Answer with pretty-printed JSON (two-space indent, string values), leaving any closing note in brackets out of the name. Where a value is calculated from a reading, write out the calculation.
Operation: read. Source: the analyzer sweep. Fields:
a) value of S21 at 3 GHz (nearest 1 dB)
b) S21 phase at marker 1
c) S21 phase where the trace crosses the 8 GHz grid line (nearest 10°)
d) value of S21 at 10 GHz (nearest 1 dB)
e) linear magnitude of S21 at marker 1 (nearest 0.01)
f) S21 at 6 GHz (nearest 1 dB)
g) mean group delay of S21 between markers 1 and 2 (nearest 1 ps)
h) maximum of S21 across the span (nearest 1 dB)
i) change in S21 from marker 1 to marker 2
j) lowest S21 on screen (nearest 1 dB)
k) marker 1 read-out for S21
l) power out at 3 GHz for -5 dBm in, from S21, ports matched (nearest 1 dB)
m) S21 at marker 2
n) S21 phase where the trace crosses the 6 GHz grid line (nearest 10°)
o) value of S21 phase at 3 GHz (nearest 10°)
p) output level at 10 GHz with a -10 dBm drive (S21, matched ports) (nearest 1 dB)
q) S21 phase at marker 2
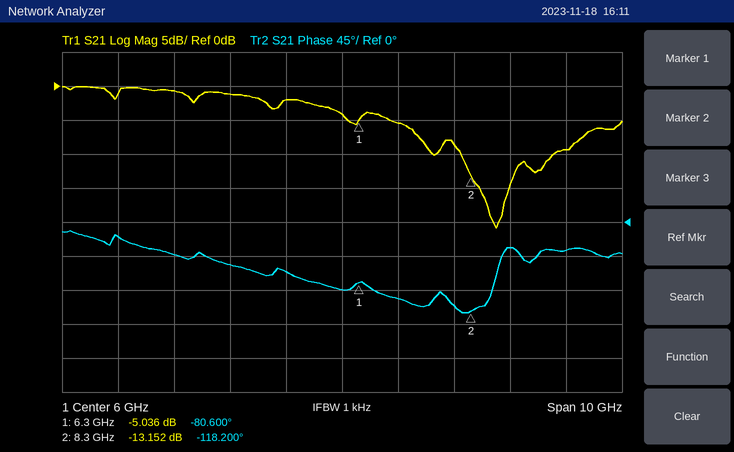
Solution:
{
  "value of S21 at 3 GHz": "-1 dB",
  "S21 phase at marker 1": "-80.600°",
  "S21 phase where the trace crosses the 8 GHz grid line": "-110°",
  "value of S21 at 10 GHz": "-9 dB",
  "linear magnitude of S21 at marker 1": "10^(-5.036/20) ≈ 0.56",
  "S21 at 6 GHz": "-4 dB",
  "mean group delay of S21 between markers 1 and 2": "−(-118.2° − (-80.6°))/(360° × 2 GHz) ≈ 52 ps",
  "maximum of S21 across the span": "0 dB",
  "change in S21 from marker 1 to marker 2": "-13.152 − (-5.036) = -8.116 dB",
  "lowest S21 on screen": "-21 dB",
  "marker 1 read-out for S21": "-5.036 dB",
  "power out at 3 GHz for -5 dBm in, from S21, ports matched": "-5 dBm + (-1 dB) = -6 dBm",
  "S21 at marker 2": "-13.152 dB",
  "S21 phase where the trace crosses the 6 GHz grid line": "-90°",
  "value of S21 phase at 3 GHz": "-40°",
  "output level at 10 GHz with a -10 dBm drive (S21, matched ports)": "-10 dBm + (-9 dB) = -19 dBm",
  "S21 phase at marker 2": "-118.200°"
}
